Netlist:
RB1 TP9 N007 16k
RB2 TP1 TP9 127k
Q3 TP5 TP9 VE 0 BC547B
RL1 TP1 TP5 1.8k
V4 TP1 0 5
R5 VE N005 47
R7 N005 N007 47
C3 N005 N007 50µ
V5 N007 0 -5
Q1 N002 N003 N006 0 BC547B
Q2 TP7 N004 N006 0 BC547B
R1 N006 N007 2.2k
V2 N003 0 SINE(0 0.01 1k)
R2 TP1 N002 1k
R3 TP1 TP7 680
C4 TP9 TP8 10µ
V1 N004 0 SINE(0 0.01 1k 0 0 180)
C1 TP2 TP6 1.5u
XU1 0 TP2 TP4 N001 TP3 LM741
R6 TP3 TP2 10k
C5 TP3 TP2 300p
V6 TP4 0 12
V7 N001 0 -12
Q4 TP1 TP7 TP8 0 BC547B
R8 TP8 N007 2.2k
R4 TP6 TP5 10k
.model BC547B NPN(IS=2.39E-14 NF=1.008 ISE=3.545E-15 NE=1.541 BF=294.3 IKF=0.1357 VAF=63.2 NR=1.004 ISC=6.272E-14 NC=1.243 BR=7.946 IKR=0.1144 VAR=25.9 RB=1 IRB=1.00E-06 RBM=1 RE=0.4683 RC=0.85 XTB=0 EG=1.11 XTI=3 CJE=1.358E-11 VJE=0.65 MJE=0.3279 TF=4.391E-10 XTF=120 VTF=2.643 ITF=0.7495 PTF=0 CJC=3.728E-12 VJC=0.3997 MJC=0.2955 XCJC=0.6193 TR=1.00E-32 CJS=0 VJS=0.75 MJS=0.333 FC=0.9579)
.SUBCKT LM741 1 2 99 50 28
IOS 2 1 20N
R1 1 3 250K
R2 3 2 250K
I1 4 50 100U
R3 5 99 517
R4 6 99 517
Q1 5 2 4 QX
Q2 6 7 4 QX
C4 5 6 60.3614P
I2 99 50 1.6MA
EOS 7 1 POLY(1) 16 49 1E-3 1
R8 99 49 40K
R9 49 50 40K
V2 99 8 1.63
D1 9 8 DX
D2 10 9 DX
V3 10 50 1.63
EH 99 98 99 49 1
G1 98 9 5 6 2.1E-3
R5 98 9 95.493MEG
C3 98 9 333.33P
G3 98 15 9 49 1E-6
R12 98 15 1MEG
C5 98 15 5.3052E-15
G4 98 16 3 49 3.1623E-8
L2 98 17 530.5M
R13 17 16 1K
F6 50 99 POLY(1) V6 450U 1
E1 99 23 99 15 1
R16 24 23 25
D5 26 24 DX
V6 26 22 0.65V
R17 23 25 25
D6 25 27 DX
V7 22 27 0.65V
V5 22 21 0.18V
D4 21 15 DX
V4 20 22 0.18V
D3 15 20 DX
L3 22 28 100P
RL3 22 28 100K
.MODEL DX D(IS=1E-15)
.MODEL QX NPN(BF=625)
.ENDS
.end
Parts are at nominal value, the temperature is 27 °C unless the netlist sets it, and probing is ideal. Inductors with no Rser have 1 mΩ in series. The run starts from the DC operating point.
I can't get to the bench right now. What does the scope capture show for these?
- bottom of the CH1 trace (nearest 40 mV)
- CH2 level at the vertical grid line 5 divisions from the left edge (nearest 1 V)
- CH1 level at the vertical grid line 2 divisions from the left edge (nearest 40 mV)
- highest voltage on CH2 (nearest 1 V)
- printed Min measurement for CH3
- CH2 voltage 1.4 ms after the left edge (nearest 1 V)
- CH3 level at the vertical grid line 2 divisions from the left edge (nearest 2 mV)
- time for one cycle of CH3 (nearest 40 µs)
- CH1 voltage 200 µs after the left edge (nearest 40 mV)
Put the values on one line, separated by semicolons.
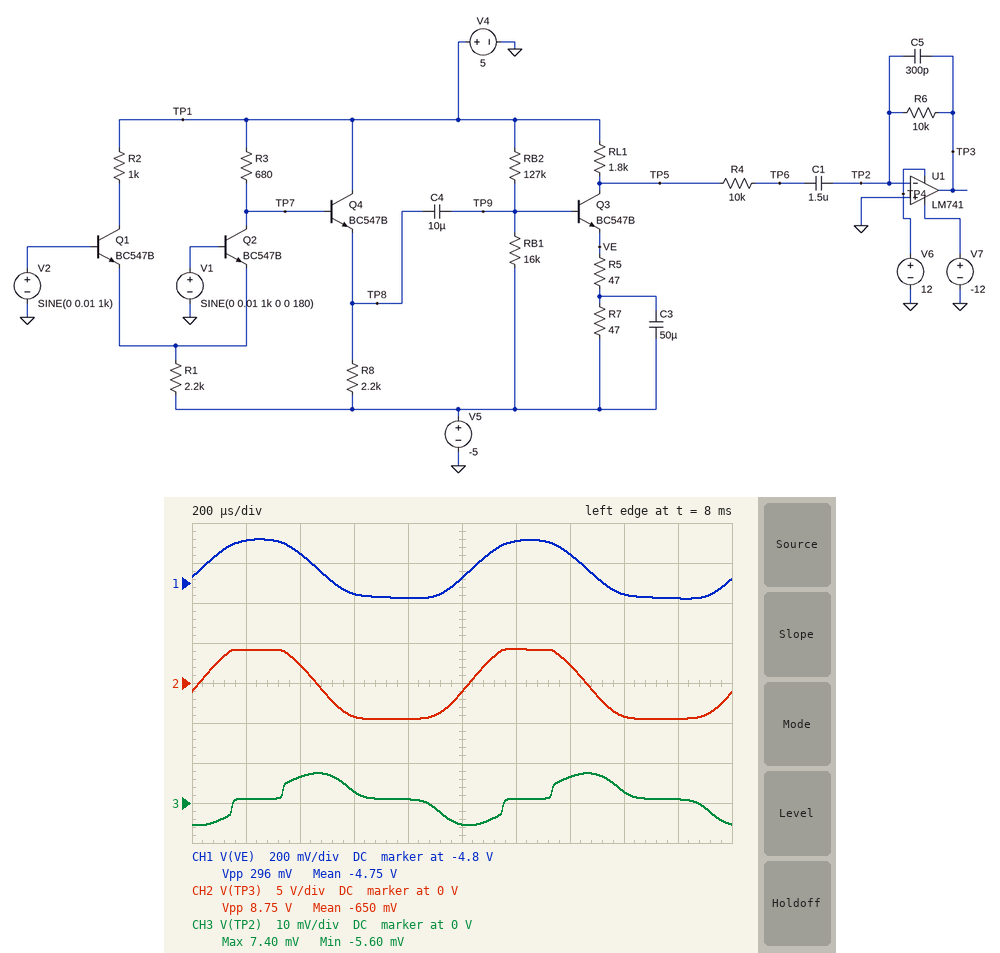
-4.88 V; -1 V; -4.64 V; 4 V; -5.60 mV; 2 V; 6 mV; 1.00 ms; -4.60 V
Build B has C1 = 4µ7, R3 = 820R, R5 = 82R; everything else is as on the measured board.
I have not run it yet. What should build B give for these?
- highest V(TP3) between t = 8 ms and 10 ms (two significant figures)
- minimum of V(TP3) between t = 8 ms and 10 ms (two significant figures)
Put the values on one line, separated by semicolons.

4.6 V; -3.8 V
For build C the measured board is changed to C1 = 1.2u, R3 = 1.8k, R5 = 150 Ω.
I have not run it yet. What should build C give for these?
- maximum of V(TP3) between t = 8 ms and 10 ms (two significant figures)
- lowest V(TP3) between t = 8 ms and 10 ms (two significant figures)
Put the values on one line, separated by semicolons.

5.2 V; -3.2 V
